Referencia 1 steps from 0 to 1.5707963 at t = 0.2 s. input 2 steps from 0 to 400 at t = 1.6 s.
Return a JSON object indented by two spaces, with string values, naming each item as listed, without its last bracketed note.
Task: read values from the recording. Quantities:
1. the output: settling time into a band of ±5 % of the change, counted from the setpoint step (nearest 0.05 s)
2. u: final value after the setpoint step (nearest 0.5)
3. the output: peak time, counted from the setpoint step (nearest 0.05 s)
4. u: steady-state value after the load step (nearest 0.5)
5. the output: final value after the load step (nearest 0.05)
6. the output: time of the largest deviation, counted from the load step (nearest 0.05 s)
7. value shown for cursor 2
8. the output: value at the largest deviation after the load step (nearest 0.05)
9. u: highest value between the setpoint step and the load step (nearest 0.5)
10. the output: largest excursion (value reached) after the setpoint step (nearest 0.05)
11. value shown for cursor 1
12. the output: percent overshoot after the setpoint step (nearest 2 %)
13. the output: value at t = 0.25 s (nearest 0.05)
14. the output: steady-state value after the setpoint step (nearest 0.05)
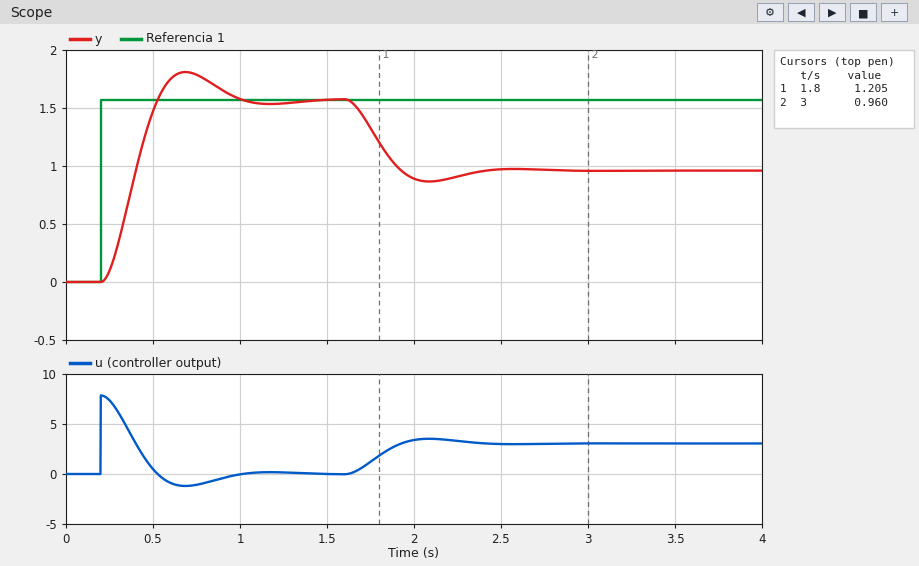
{
  "the output: settling time into a band of ±5 % of the change, counted from the setpoint step": "0.70 s",
  "u: final value after the setpoint step": "0.0",
  "the output: peak time, counted from the setpoint step": "0.50 s",
  "u: steady-state value after the load step": "3.0",
  "the output: final value after the load step": "0.95",
  "the output: time of the largest deviation, counted from the load step": "0.50 s",
  "value shown for cursor 2": "0.960",
  "the output: value at the largest deviation after the load step": "0.85",
  "u: highest value between the setpoint step and the load step": "8.0",
  "the output: largest excursion (value reached) after the setpoint step": "1.80",
  "value shown for cursor 1": "1.205",
  "the output: percent overshoot after the setpoint step": "16 %",
  "the output: value at t = 0.25 s": "0.10",
  "the output: steady-state value after the setpoint step": "1.55"
}
